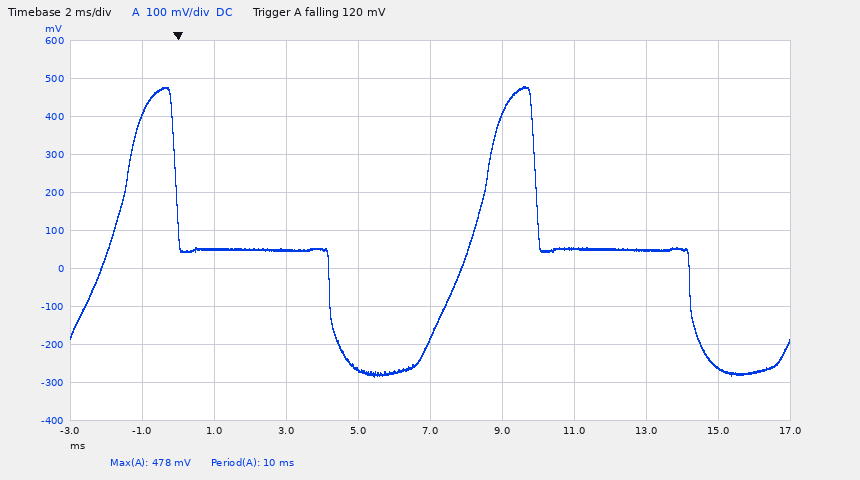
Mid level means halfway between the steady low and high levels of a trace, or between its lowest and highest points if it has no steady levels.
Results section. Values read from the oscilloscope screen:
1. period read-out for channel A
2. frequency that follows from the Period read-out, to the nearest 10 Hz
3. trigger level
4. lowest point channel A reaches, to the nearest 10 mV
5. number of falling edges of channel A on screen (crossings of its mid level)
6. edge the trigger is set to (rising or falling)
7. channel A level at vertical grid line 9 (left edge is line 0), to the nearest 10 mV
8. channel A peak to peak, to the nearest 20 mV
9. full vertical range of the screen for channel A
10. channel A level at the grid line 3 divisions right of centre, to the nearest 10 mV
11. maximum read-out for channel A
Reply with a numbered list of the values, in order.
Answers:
1. 10 ms
2. 100 Hz
3. 120 mV
4. -280 mV
5. 2
6. falling
7. -260 mV
8. 760 mV
9. 1 V
10. 50 mV
11. 478 mV
